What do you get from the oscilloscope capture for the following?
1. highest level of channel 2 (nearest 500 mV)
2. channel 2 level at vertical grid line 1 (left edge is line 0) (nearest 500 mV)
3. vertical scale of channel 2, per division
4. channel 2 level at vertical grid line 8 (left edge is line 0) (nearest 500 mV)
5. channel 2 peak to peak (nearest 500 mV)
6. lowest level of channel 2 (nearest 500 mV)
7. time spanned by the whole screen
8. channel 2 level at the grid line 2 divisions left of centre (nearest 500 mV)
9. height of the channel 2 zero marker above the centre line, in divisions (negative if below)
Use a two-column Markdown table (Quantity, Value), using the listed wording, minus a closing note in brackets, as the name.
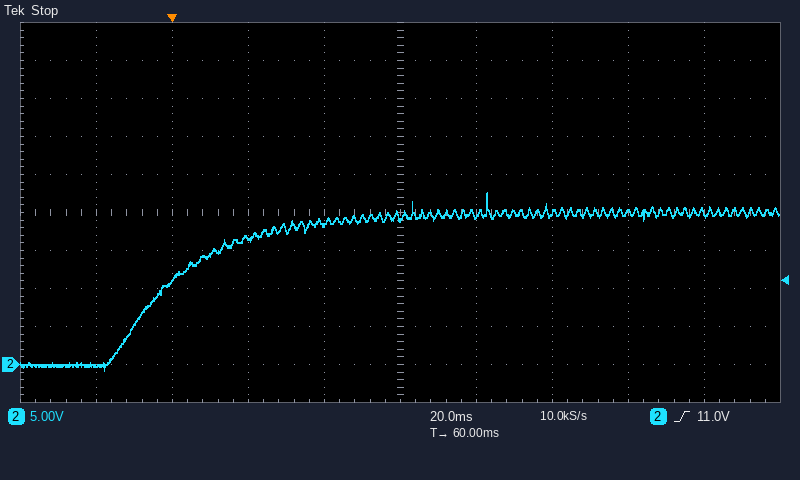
| Quantity | Value |
|---|---|
| highest level of channel 2 | 22.5 V |
| channel 2 level at vertical grid line 1 (left edge is line 0) | 0.0 V |
| vertical scale of channel 2, per division | 5 V |
| channel 2 level at vertical grid line 8 (left edge is line 0) | 20.0 V |
| channel 2 peak to peak | 23.5 V |
| lowest level of channel 2 | -1.0 V |
| time spanned by the whole screen | 200 ms |
| channel 2 level at the grid line 2 divisions left of centre | 16.5 V |
| height of the channel 2 zero marker above the centre line, in divisions | -4.0 div |
